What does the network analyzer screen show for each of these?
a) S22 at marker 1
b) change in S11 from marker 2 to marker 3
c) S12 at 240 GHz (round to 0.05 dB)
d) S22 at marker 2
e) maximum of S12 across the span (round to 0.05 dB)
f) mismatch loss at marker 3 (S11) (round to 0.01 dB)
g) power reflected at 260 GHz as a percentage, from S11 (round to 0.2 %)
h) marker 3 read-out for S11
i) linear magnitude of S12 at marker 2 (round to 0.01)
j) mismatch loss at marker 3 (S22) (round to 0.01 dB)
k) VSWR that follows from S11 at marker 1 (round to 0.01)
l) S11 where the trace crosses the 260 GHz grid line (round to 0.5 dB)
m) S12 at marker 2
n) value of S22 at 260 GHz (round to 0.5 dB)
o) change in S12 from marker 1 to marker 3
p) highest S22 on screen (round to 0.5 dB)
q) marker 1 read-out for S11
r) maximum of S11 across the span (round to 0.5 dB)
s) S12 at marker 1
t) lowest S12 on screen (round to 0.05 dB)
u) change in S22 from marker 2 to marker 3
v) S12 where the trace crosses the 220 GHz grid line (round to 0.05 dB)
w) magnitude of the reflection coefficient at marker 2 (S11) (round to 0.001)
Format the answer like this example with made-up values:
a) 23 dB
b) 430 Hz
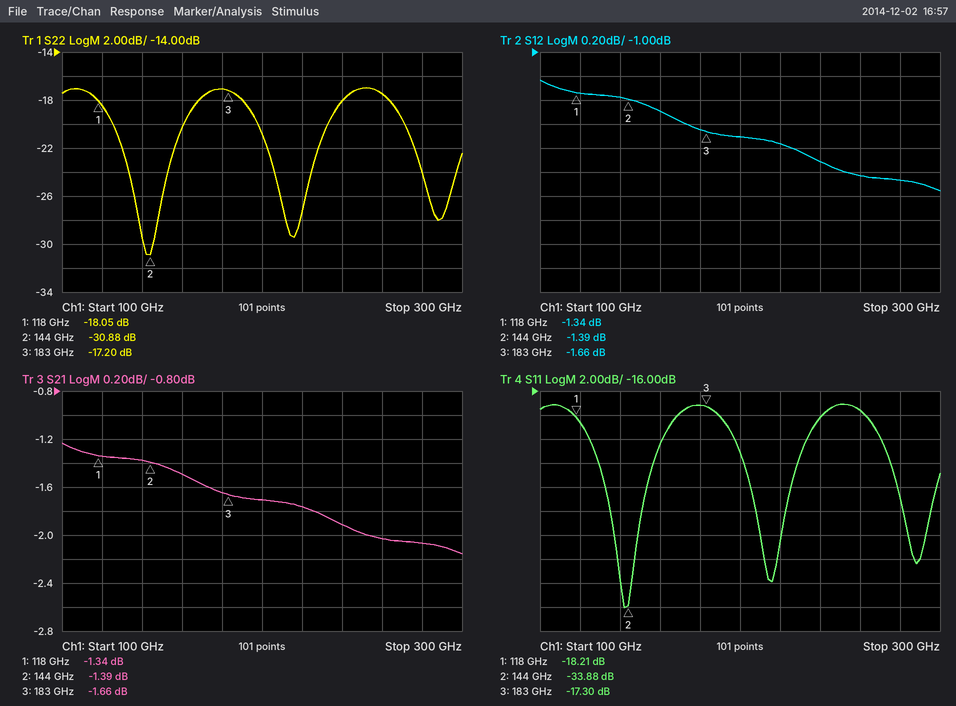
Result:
a) -18.05 dB
b) 16.58 dB
c) -1.90 dB
d) -30.88 dB
e) -1.25 dB
f) 0.08 dB
g) 1.8 %
h) -17.30 dB
i) 0.85
j) 0.08 dB
k) 1.28
l) -17.5 dB
m) -1.39 dB
n) -17.5 dB
o) -0.32 dB
p) -17.0 dB
q) -18.21 dB
r) -17.0 dB
s) -1.34 dB
t) -2.15 dB
u) 13.68 dB
v) -1.75 dB
w) 0.020
